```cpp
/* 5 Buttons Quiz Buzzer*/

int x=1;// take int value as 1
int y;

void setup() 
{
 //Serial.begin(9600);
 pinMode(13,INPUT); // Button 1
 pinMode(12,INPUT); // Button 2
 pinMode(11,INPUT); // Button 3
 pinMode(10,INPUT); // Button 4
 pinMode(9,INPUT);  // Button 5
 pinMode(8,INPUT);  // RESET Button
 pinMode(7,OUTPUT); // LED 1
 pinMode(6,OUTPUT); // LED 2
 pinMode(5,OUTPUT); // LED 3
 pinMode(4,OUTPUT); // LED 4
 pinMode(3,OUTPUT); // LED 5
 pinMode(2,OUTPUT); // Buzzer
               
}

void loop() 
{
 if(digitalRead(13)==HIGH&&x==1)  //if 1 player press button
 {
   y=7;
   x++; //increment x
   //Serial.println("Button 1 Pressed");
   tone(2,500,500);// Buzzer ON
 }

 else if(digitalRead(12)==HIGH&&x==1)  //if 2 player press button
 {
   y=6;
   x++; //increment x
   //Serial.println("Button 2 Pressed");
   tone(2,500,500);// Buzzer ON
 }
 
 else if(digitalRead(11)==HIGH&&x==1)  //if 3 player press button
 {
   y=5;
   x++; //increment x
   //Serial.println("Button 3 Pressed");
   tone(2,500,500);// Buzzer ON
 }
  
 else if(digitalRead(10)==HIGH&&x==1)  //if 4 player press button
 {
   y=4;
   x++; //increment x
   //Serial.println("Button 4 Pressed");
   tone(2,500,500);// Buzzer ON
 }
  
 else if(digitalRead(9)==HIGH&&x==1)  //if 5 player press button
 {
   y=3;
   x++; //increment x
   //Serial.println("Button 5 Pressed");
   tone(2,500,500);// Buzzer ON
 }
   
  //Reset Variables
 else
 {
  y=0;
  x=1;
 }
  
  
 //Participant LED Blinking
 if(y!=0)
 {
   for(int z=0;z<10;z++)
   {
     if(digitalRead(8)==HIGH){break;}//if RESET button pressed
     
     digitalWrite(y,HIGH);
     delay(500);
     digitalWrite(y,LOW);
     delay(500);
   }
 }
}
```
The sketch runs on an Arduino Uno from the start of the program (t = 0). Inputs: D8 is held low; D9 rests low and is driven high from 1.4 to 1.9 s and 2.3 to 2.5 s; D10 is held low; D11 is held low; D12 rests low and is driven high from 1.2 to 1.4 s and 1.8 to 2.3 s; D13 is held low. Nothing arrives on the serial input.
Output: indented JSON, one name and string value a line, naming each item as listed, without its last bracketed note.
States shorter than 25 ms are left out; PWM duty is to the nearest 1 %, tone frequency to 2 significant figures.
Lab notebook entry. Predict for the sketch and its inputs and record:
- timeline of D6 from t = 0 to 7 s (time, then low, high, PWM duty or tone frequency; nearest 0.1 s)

{
  "timeline of D6 from t = 0 to 7 s": "0 s low; 1.2 s high; 1.7 s low; 2.2 s high; 2.7 s low; 3.2 s high; 3.7 s low; 4.2 s high; 4.7 s low; 5.2 s high; 5.7 s low; 6.2 s high; 6.7 s low"
}
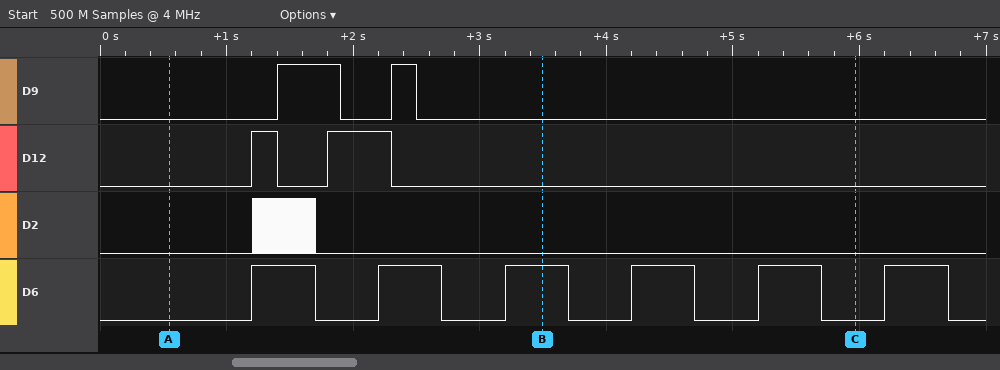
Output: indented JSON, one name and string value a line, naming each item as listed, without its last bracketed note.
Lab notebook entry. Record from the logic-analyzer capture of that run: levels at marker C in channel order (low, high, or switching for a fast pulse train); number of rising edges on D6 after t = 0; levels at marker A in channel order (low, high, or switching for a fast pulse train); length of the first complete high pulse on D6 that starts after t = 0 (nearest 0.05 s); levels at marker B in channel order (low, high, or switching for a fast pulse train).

{
  "levels at marker C in channel order": "D9 low, D12 low, D2 low, D6 low",
  "number of rising edges on D6 after t = 0": "6",
  "levels at marker A in channel order": "D9 low, D12 low, D2 low, D6 low",
  "length of the first complete high pulse on D6 that starts after t = 0": "0.50 s",
  "levels at marker B in channel order": "D9 low, D12 low, D2 low, D6 high"
}
